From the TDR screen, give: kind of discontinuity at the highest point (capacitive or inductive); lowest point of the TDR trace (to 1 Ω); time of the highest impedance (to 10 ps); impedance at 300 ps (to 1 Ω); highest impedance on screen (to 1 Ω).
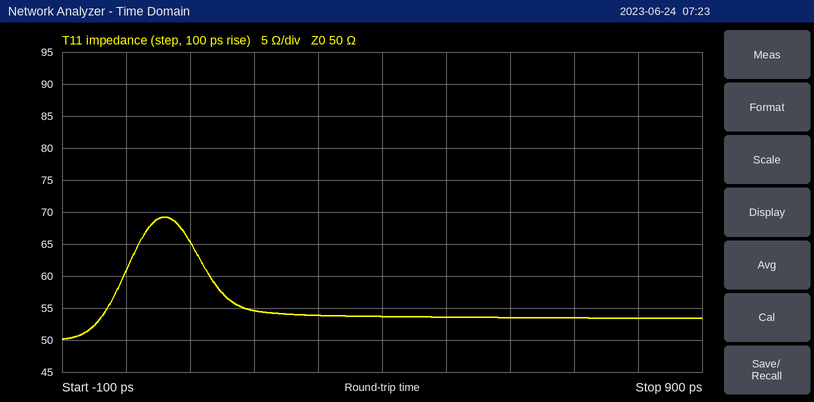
inductive
50 Ω
60 ps
54 Ω
69 Ω
